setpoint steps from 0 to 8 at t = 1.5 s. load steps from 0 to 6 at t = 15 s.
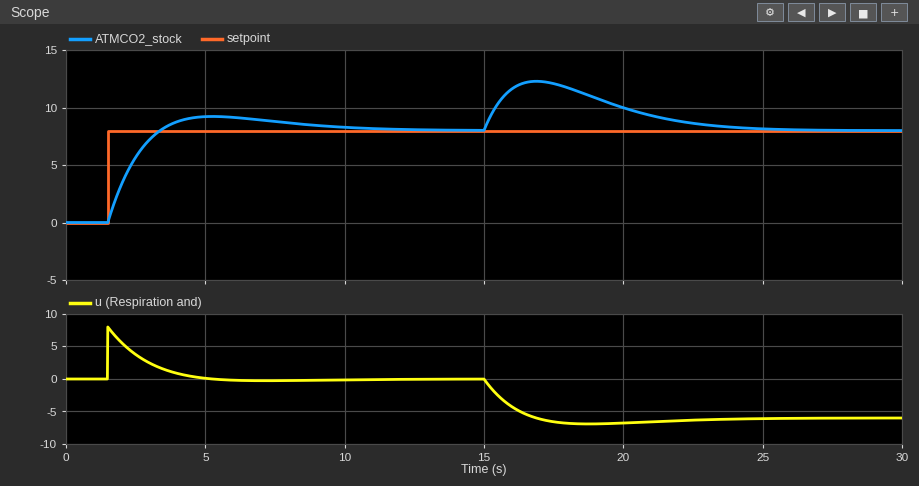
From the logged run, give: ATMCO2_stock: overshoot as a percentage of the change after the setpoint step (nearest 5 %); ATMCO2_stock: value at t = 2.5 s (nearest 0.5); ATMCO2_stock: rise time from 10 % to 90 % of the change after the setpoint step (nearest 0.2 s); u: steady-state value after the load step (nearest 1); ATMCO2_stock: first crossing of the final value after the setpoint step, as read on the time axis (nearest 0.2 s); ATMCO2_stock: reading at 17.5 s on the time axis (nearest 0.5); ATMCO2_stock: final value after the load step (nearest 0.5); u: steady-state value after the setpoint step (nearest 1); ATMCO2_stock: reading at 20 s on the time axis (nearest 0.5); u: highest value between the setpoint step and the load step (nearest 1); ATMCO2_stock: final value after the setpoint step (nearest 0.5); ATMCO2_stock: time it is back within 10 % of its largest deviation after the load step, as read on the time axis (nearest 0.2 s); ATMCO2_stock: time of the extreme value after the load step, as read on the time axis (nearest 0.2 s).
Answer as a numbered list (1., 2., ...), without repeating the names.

1. 15 %
2. 5.5
3. 1.4 s
4. -6
5. 3.4 s
6. 12.0
7. 8.0
8. 0
9. 10.0
10. 8
11. 8.0
12. 23.2 s
13. 16.8 s
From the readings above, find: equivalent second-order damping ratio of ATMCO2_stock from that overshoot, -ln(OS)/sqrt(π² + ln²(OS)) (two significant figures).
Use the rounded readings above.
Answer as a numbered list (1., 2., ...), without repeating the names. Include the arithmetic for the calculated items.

1. ln(0.15) = -1.897; 1.897 / sqrt(9.870 + 3.599) = 0.52
